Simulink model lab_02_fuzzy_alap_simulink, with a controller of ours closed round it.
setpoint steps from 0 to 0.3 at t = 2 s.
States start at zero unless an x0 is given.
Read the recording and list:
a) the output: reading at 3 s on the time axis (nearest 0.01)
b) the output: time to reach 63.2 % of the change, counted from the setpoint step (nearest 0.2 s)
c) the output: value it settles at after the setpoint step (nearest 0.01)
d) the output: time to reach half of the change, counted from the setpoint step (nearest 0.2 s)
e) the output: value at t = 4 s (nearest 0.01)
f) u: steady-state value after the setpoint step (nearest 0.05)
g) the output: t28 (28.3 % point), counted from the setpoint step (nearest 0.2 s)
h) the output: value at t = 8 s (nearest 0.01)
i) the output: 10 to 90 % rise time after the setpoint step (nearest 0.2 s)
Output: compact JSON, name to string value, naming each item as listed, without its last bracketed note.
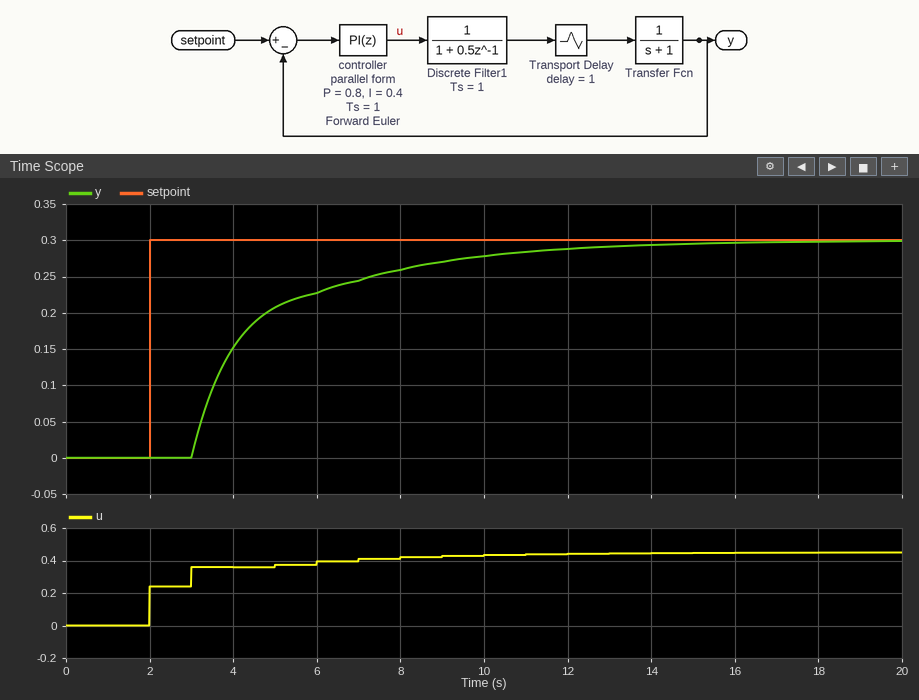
{"the output: reading at 3 s on the time axis": "0.00", "the output: time to reach 63.2 % of the change, counted from the setpoint step": "2.6 s", "the output: value it settles at after the setpoint step": "0.30", "the output: time to reach half of the change, counted from the setpoint step": "2.0 s", "the output: value at t = 4 s": "0.15", "u: steady-state value after the setpoint step": "0.45", "the output: t28 (28.3 % point), counted from the setpoint step": "1.4 s", "the output: value at t = 8 s": "0.26", "the output: 10 to 90 % rise time after the setpoint step": "5.8 s"}
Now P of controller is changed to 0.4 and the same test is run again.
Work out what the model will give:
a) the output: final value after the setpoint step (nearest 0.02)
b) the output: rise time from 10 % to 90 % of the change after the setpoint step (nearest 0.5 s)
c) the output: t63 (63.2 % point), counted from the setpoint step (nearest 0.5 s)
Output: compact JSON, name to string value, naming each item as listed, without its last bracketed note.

{"the output: final value after the setpoint step": "0.30", "the output: rise time from 10 % to 90 % of the change after the setpoint step": "4.5 s", "the output: t63 (63.2 % point), counted from the setpoint step": "3.5 s"}
